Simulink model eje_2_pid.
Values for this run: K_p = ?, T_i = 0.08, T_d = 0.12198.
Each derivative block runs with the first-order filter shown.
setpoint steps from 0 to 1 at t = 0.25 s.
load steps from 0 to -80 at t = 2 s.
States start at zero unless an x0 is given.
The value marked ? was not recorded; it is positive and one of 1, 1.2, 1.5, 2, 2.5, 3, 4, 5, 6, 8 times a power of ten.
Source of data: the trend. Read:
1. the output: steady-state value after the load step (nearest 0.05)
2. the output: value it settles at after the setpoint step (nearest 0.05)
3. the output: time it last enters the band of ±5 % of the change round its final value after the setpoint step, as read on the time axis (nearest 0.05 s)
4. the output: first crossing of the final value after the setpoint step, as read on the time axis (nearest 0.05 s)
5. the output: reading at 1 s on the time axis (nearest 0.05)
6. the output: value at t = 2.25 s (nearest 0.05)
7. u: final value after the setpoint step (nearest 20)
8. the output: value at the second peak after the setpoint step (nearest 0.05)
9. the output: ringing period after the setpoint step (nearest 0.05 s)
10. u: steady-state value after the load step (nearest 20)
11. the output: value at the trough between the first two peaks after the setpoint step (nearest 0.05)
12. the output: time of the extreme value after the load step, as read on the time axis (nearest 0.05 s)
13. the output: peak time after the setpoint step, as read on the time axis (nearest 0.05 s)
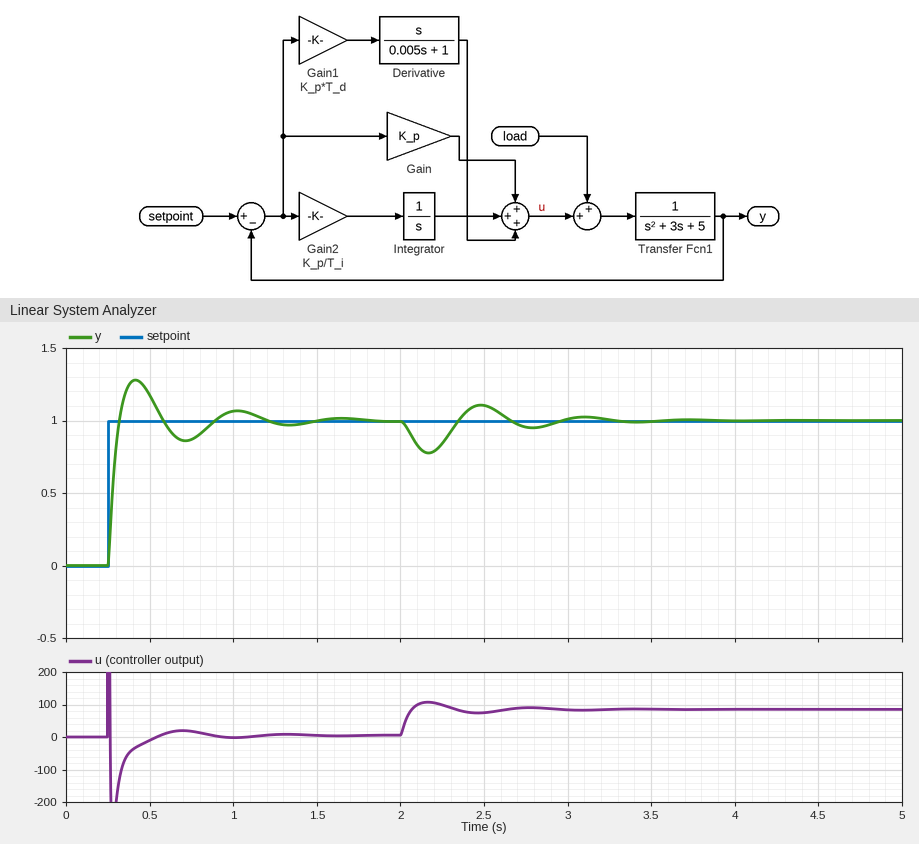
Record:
1.00
1.00
1.10 s
0.30 s
1.05
0.85
0
1.05
0.60 s
80
0.85
2.15 s
0.40 s
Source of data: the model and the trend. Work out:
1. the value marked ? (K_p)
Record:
200
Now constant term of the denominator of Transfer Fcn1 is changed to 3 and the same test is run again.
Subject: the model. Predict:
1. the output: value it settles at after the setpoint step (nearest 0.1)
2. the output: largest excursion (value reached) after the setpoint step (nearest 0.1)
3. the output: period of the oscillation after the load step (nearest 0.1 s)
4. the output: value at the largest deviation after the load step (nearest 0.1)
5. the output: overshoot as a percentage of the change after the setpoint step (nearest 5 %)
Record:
1.0
1.3
0.6 s
0.8
30 %
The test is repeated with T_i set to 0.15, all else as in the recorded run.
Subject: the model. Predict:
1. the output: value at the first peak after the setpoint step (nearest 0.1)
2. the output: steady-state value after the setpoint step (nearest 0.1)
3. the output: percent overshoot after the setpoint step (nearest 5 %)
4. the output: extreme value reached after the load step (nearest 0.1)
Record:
1.2
1.0
20 %
0.7
